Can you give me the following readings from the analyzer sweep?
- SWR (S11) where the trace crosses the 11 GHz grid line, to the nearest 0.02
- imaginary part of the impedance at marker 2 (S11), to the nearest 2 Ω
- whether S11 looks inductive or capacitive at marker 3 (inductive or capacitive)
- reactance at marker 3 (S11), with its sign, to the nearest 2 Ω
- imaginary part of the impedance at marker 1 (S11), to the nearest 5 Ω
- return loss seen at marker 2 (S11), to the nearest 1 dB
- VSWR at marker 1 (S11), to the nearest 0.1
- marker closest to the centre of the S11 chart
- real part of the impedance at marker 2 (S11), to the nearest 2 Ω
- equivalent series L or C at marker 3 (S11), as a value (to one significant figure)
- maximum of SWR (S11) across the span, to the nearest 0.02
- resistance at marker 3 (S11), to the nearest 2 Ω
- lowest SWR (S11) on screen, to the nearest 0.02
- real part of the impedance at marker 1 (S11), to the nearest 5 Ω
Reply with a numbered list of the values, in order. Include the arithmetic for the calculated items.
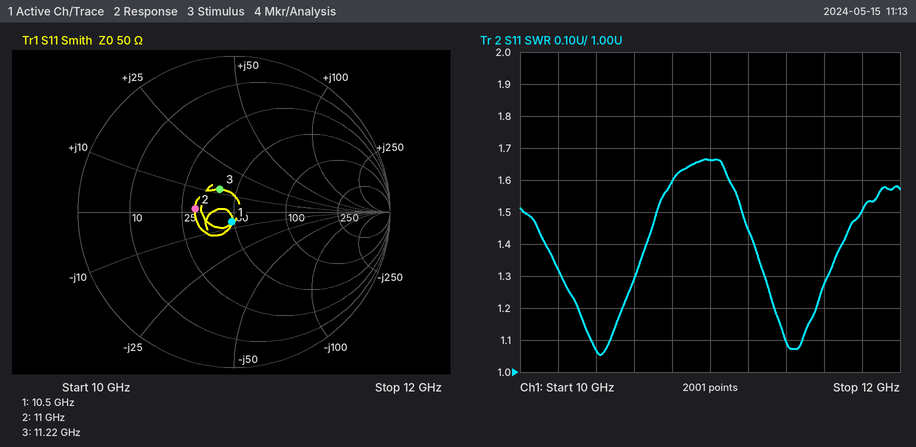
1. 1.66
2. +2 Ω
3. inductive
4. +12 Ω
5. -5 Ω
6. 12 dB
7. 1.1
8. marker 1
9. 30 Ω
10. L = 12 Ω/(2π × 11.22 GHz) ≈ 170 pH, so 200 pH to one significant figure
11. 1.66
12. 40 Ω
13. 1.06
14. 50 Ω
